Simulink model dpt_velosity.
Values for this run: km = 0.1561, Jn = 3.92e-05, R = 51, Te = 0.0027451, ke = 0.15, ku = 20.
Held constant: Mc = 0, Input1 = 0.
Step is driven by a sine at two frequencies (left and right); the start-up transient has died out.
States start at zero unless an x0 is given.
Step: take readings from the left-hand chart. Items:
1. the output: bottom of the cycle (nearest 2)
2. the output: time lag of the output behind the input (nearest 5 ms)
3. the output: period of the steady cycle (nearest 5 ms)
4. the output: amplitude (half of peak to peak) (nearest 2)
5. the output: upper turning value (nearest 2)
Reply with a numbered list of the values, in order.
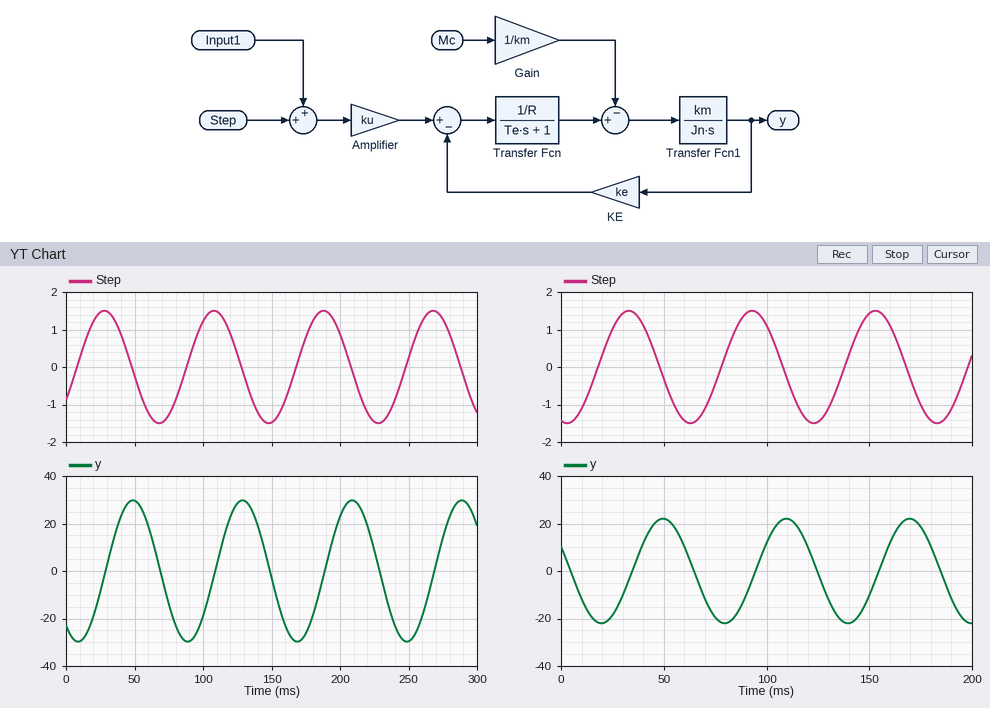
1. -30
2. 20 ms
3. 80 ms
4. 30
5. 30
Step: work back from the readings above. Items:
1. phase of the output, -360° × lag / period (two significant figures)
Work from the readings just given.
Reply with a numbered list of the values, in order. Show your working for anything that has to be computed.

1. -360 × 20 / 80 = -90°
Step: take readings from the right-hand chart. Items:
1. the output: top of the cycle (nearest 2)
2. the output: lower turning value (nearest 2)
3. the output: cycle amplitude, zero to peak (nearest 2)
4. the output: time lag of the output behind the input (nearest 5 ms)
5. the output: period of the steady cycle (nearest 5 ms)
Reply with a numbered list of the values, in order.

1. 22
2. -22
3. 22
4. 15 ms
5. 60 ms
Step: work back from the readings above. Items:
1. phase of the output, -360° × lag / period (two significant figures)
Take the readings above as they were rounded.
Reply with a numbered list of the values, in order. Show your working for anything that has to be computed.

1. -360 × 15 / 60 = -90°
